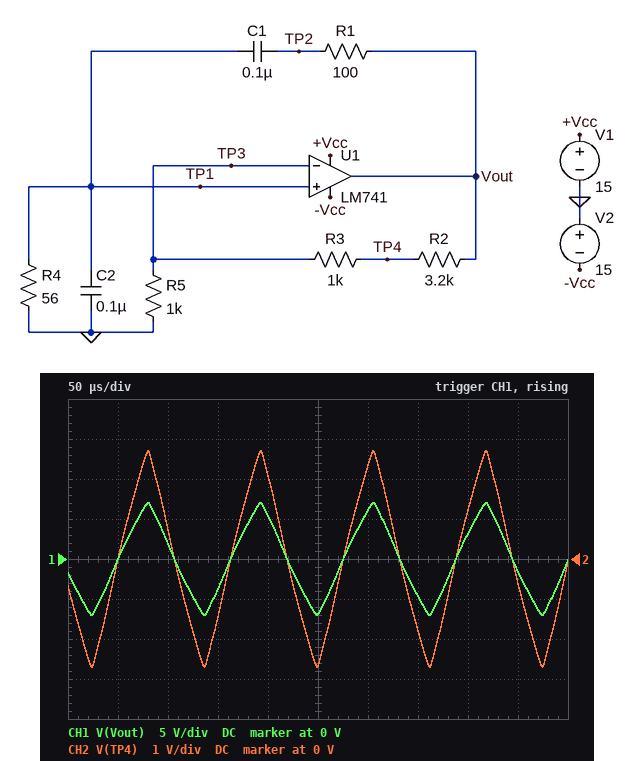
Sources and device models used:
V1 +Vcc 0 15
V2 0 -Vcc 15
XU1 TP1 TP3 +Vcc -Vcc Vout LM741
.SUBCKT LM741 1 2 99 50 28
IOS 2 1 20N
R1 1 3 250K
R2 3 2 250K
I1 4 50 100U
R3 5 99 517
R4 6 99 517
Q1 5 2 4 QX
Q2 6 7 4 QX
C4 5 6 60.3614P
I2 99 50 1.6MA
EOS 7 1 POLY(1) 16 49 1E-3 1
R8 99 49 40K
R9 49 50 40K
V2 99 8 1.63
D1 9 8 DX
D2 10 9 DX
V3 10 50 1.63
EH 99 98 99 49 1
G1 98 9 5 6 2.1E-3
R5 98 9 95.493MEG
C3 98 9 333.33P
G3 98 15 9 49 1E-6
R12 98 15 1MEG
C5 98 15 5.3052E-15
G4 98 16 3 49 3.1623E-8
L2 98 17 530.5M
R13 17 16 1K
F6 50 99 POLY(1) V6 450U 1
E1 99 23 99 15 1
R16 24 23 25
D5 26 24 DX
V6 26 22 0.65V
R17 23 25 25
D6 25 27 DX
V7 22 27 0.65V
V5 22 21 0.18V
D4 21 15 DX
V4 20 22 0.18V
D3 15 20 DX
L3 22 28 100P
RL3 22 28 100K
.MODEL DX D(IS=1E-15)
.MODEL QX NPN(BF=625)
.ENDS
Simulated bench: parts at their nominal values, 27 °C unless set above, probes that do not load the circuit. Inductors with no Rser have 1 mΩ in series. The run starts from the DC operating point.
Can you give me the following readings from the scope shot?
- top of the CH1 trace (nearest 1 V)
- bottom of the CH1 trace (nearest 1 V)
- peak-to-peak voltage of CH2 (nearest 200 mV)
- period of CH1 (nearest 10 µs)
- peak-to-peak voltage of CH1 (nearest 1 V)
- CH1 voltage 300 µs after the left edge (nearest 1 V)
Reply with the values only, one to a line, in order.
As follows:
7 V
-7 V
5.4 V
110 µs
14 V
6 V
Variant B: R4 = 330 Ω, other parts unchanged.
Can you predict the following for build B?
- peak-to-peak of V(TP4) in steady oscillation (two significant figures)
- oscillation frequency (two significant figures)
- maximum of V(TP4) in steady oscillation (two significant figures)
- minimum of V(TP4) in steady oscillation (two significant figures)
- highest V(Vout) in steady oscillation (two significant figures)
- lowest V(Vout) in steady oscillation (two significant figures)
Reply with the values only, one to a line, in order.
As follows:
11 V
3.1 kHz
5.3 V
-5.3 V
14 V
-14 V
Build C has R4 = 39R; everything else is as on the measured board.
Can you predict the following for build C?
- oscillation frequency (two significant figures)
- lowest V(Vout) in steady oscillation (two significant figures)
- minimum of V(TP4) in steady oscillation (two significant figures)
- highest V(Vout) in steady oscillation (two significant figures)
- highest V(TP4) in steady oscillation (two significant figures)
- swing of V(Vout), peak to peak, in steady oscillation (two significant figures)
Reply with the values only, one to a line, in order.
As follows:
14 kHz
-4.2 V
-1.6 V
4.2 V
1.6 V
8.5 V
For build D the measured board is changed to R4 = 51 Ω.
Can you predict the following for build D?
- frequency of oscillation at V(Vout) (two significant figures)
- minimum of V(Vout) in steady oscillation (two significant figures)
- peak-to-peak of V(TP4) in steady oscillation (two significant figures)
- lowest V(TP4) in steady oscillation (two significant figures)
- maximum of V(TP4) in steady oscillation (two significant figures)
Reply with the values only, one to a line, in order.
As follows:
10 kHz
-6.2 V
4.8 V
-2.4 V
2.4 V
